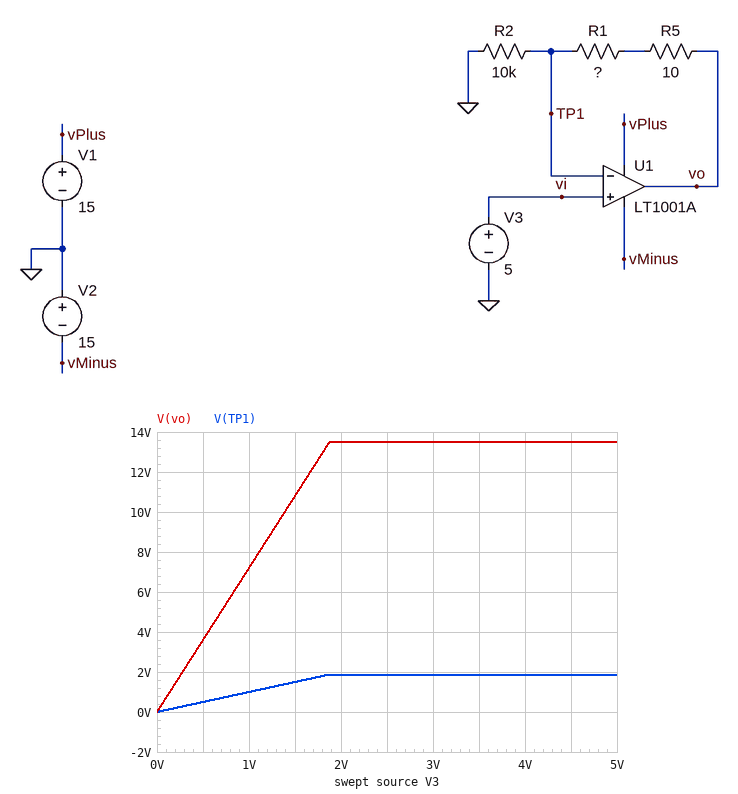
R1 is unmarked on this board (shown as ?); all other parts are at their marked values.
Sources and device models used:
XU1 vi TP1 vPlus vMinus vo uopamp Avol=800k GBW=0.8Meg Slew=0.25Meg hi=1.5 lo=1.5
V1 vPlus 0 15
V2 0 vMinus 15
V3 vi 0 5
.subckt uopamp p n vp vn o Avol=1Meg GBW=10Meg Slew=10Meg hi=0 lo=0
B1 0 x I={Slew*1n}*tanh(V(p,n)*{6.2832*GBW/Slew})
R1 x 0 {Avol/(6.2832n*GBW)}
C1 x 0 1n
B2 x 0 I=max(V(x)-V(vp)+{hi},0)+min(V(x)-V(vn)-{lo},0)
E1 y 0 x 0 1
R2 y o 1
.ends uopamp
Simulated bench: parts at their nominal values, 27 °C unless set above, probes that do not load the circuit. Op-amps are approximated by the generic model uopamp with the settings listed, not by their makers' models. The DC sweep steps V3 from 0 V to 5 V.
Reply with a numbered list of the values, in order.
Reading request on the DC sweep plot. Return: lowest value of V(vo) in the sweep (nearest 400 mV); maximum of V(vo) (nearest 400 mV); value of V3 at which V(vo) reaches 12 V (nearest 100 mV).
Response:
1. 0 V
2. 13.6 V
3. 1.7 V
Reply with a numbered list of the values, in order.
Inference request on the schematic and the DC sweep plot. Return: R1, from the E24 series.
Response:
1. 62 kΩ
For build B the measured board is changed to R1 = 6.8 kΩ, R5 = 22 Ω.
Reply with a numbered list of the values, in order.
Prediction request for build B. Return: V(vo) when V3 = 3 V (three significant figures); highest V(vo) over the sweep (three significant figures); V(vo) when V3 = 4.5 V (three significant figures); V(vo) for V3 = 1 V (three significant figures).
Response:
1. 5.05 V
2. 8.41 V
3. 7.57 V
4. 1.68 V
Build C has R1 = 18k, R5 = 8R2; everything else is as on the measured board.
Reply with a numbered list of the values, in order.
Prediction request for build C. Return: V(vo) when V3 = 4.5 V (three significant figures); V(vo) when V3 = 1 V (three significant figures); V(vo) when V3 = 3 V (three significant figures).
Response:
1. 12.6 V
2. 2.80 V
3. 8.40 V
